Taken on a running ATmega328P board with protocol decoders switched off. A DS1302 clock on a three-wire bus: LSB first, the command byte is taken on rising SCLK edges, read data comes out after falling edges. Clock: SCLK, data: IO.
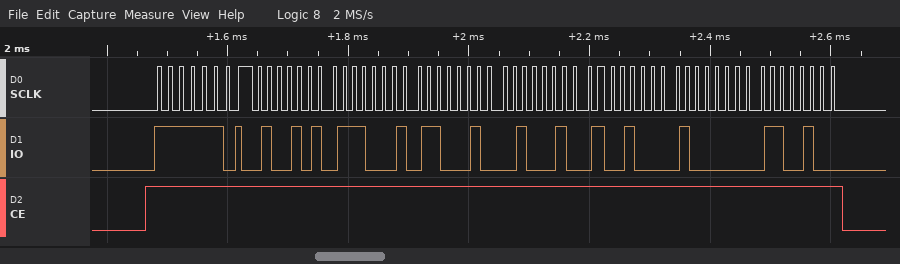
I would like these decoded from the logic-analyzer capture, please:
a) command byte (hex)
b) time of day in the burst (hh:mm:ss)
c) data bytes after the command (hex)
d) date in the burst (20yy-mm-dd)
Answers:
0xBF
23:47:52
52 47 23 22 09 01 13
2013-09-22
